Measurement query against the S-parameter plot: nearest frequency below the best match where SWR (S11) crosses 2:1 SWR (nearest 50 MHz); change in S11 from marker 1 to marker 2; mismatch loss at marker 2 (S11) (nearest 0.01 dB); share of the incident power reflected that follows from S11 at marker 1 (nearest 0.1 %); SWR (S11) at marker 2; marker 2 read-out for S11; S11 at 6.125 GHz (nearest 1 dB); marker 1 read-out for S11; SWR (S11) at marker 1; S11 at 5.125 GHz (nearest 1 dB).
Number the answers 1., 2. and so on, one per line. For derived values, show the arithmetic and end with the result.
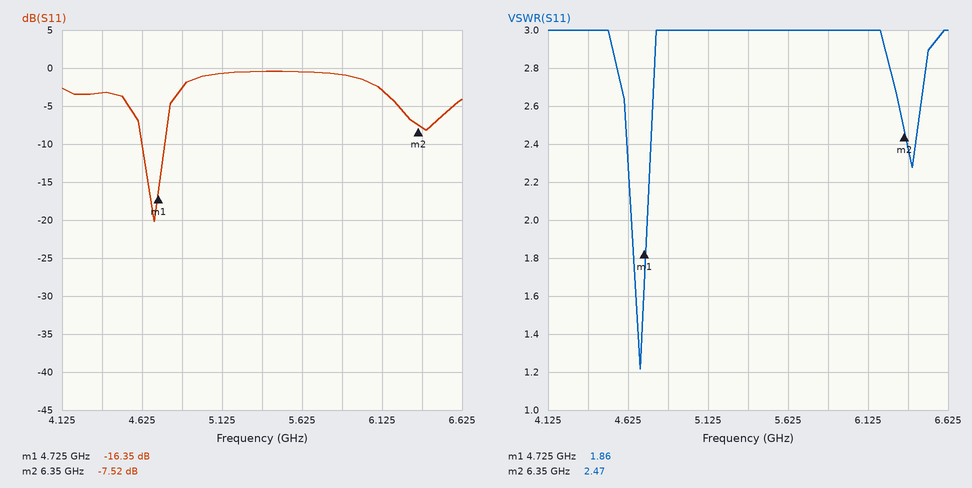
1. 4.65 GHz
2. -7.52 − (-16.35) = 8.83 dB
3. −10 log10(1 − 10^(-7.52/10)) ≈ 0.85 dB
4. 10^(-16.35/10) ≈ 2.3 %
5. 2.47
6. -7.52 dB
7. -3 dB
8. -16.35 dB
9. 1.86
10. -1 dB
